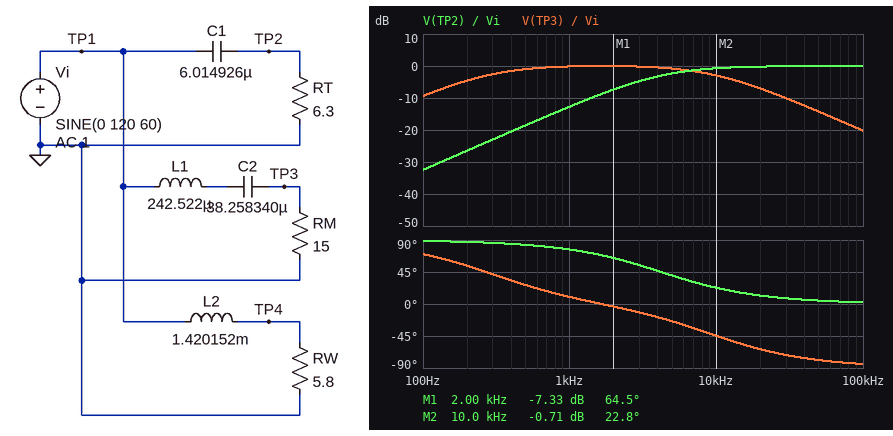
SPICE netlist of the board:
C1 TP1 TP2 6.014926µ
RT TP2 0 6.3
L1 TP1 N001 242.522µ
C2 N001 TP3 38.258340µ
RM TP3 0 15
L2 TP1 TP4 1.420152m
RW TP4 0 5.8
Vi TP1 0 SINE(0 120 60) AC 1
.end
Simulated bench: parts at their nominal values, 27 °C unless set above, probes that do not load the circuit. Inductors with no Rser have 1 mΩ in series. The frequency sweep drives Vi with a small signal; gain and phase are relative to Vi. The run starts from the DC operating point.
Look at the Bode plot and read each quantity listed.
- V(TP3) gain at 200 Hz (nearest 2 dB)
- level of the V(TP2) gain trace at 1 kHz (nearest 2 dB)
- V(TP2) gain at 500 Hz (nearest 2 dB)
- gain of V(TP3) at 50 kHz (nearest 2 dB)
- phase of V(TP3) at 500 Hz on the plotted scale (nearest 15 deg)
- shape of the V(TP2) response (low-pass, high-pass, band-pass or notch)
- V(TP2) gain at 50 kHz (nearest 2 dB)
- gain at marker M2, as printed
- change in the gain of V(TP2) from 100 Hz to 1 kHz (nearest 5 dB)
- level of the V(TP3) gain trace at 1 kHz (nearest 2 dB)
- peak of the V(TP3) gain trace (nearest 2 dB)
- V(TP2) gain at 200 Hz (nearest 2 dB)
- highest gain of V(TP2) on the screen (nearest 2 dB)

-4 dB
-12 dB
-18 dB
-14 dB
30 deg
high-pass
0 dB
-0.71 dB
20 dB
0 dB
0 dB
-26 dB
0 dB
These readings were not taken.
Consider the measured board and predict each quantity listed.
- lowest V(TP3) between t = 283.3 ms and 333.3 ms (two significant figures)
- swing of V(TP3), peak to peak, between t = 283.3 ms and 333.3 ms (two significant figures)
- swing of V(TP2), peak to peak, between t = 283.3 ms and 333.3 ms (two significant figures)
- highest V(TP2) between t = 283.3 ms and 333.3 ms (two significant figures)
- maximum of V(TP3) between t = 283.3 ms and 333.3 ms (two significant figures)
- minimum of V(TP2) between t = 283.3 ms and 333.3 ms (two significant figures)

-25 V
51 V
3.4 V
1.7 V
25 V
-1.7 V
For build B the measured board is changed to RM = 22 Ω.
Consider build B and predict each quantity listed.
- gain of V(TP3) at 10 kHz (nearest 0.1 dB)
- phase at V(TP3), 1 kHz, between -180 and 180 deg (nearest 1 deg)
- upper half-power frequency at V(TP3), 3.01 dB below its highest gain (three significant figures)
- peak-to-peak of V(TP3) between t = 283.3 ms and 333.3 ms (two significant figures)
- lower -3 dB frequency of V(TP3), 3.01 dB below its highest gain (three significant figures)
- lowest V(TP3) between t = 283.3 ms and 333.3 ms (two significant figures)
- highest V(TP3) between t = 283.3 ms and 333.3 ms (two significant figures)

-1.6 dB
7 deg
14.6 kHz
73 V
187 Hz
-36 V
36 V
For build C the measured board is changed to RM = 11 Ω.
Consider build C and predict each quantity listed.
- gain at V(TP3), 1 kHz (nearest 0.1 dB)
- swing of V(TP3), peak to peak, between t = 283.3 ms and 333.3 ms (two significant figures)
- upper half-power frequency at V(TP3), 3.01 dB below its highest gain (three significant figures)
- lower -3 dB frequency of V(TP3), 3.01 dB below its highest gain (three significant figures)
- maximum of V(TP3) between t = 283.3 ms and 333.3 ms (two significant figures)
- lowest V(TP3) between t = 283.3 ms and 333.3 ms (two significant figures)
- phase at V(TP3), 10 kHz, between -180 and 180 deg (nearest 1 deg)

-0.2 dB
38 V
7.58 kHz
360 Hz
19 V
-19 V
-53 deg
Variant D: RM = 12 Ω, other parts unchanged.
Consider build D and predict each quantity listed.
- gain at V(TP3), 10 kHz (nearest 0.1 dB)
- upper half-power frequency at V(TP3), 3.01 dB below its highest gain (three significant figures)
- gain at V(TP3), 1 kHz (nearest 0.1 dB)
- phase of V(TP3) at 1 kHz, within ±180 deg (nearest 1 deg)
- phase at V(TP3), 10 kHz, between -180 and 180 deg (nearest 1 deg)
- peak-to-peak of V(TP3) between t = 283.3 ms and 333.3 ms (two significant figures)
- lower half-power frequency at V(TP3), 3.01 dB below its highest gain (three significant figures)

-4.0 dB
8.21 kHz
-0.2 dB
12 deg
-51 deg
41 V
333 Hz
